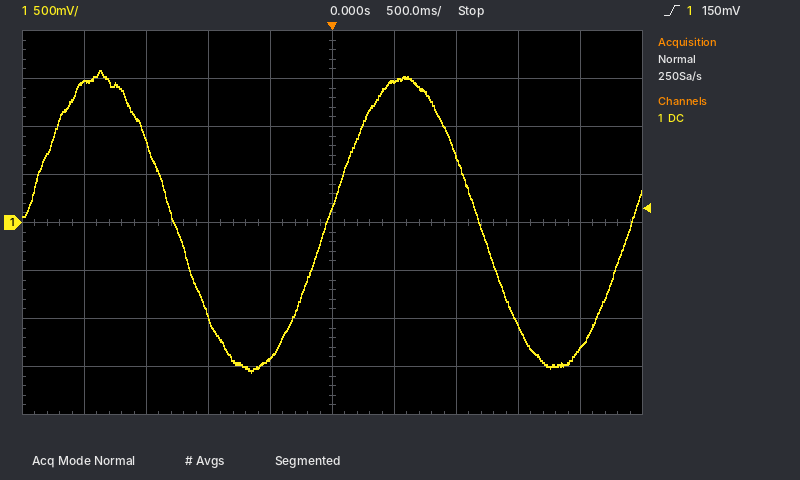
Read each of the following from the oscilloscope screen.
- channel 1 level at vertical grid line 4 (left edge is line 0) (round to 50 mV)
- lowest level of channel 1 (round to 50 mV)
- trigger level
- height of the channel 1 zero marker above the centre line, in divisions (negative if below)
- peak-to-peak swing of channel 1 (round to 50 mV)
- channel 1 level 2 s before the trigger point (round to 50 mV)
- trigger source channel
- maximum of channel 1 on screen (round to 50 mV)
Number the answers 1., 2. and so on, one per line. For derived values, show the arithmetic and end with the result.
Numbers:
1. -1.40 V
2. -1.55 V
3. 150 mV
4. 0.0 div
5. 1.60 V − (-1.55 V) = 3.15 V
6. 1.45 V
7. channel 1
8. 1.60 V
